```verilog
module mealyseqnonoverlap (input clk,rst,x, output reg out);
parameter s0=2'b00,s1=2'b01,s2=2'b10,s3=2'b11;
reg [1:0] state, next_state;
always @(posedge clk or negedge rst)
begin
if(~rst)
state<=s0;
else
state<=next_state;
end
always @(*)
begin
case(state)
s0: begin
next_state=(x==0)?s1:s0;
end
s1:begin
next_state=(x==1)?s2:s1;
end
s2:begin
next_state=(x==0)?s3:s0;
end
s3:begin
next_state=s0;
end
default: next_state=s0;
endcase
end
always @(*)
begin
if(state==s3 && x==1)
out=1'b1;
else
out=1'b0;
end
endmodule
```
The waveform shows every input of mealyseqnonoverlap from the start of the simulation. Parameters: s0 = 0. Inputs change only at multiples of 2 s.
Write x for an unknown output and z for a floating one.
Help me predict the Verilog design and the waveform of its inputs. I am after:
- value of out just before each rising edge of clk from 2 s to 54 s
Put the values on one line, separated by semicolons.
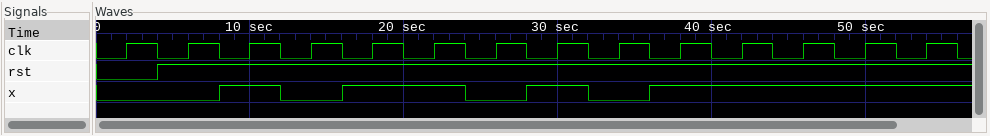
0 0 0 0 1 0 0 0 0 1 0 0 0 0
